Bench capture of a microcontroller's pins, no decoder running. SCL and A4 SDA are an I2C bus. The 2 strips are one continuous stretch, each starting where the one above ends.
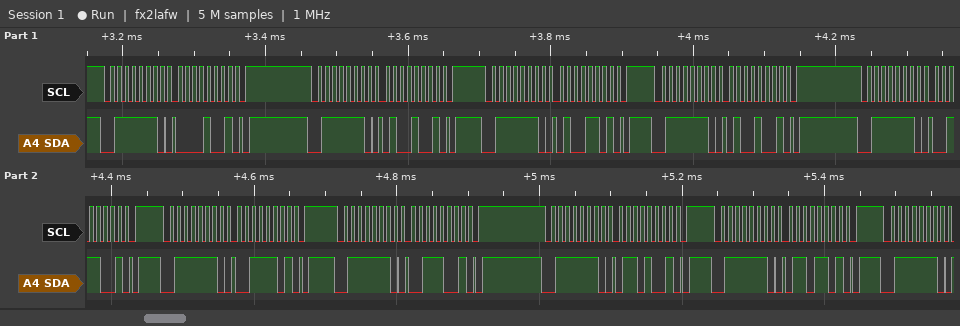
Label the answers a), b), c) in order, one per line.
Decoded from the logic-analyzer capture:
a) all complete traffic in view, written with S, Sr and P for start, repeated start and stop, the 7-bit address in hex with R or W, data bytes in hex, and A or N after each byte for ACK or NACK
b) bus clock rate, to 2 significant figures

a) S 3FW A 09 A P S 3FW A 49 A P S 3FW A 4D A P S 3FW A 49 A P S 3FW A 39 A P S 3FW A 3D A P S 3FW A 39 A P S 3FW A 69 A P S 3FW A 6D A P S 3FW A
b) 100 kHz
